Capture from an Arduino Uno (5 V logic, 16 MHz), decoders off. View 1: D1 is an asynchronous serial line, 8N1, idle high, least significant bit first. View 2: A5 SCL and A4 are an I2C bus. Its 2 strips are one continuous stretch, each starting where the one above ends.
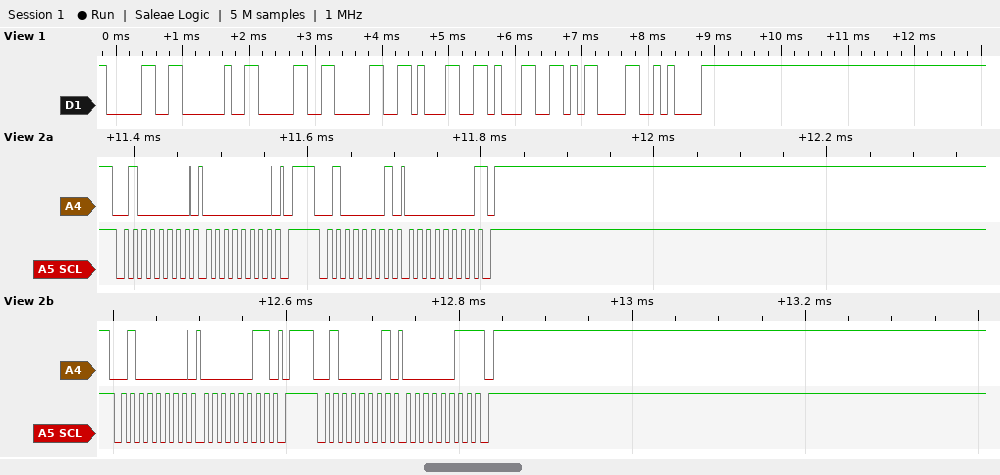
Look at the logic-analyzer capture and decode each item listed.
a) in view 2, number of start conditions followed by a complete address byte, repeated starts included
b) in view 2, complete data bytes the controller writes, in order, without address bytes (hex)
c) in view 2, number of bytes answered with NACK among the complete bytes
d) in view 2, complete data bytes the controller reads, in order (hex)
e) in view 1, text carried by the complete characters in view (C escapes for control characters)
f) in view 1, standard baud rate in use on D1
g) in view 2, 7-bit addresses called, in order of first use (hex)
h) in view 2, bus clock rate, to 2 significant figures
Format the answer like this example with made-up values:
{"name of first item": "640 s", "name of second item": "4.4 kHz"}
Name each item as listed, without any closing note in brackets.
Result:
{"in view 2, number of start conditions followed by a complete address byte, repeated starts included": "4", "in view 2, complete data bytes the controller writes, in order, without address bytes": "00 03", "in view 2, number of bytes answered with NACK among the complete bytes": "2", "in view 2, complete data bytes the controller reads, in order": "00 03", "in view 1, text carried by the complete characters in view": "\"0 0011\\r\\n\"", "in view 1, standard baud rate in use on D1": "9600 baud", "in view 2, 7-bit addresses called, in order of first use": "0x20", "in view 2, bus clock rate, to 2 significant figures": "100 kHz"}
